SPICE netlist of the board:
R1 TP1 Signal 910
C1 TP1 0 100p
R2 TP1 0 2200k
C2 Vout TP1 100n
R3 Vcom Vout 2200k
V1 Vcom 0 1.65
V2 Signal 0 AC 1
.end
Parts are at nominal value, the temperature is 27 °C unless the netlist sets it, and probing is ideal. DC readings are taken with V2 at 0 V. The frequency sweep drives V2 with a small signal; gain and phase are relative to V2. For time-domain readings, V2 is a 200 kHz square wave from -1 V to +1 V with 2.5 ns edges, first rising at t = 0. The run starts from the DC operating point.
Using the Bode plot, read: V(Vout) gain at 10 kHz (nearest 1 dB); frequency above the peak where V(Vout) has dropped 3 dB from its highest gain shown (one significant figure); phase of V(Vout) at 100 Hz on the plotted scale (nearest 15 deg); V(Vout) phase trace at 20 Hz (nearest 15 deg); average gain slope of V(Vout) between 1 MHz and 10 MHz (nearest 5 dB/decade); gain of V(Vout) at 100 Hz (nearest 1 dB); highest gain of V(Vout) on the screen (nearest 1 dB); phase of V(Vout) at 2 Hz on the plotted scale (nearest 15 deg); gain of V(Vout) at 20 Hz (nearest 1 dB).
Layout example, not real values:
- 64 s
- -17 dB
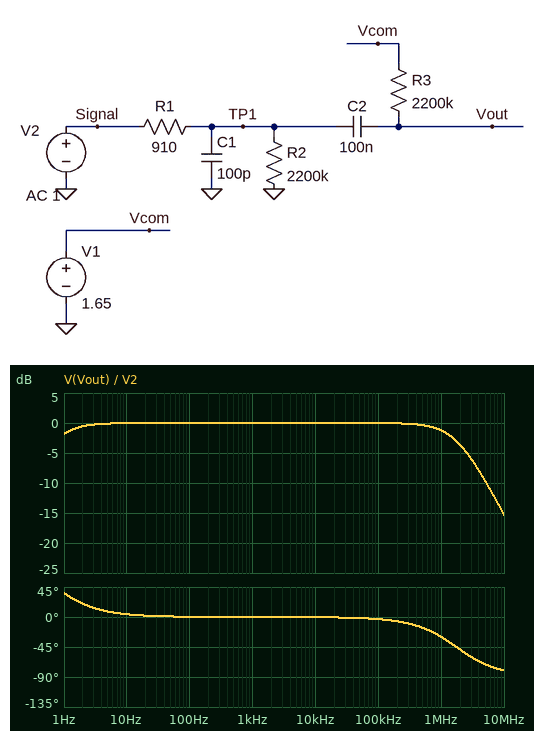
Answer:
- 0 dB
- 2 MHz
- 0 deg
- 0 deg
- -15 dB/decade
- 0 dB
- 0 dB
- 15 deg
- 0 dB
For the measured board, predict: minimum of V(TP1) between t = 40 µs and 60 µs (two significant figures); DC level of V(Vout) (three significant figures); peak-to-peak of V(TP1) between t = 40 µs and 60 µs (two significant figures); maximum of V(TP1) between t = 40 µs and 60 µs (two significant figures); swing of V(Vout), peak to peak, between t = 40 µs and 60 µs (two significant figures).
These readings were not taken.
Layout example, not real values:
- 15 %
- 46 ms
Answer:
- -1.0 V
- 1.65 V
- 2.0 V
- 1.0 V
- 2.0 V
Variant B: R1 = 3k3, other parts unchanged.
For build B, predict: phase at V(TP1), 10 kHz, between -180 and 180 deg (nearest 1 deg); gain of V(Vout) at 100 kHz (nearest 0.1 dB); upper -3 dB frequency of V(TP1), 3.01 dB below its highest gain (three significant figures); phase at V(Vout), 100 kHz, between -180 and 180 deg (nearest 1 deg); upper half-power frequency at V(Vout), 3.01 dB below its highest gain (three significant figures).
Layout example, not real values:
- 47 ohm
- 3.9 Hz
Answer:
- -1 deg
- -0.2 dB
- 482 kHz
- -12 deg
- 484 kHz
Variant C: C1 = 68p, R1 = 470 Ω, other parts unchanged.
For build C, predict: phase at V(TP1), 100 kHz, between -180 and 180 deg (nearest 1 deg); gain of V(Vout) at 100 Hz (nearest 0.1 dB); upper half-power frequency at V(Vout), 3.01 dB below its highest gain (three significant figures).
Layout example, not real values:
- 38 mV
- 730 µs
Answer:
- -1 deg
- 0 dB
- 4.98 MHz
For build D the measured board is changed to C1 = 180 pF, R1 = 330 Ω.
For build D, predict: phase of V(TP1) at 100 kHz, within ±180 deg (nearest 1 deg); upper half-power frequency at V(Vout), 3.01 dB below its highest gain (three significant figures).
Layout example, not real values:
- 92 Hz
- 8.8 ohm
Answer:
- -2 deg
- 2.68 MHz
